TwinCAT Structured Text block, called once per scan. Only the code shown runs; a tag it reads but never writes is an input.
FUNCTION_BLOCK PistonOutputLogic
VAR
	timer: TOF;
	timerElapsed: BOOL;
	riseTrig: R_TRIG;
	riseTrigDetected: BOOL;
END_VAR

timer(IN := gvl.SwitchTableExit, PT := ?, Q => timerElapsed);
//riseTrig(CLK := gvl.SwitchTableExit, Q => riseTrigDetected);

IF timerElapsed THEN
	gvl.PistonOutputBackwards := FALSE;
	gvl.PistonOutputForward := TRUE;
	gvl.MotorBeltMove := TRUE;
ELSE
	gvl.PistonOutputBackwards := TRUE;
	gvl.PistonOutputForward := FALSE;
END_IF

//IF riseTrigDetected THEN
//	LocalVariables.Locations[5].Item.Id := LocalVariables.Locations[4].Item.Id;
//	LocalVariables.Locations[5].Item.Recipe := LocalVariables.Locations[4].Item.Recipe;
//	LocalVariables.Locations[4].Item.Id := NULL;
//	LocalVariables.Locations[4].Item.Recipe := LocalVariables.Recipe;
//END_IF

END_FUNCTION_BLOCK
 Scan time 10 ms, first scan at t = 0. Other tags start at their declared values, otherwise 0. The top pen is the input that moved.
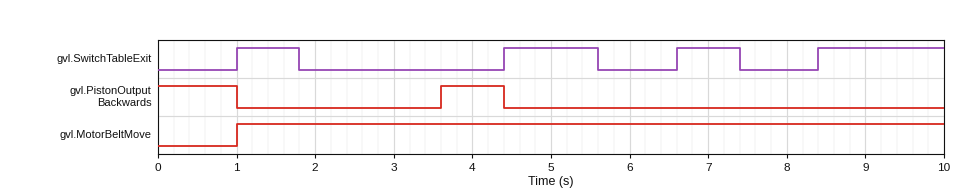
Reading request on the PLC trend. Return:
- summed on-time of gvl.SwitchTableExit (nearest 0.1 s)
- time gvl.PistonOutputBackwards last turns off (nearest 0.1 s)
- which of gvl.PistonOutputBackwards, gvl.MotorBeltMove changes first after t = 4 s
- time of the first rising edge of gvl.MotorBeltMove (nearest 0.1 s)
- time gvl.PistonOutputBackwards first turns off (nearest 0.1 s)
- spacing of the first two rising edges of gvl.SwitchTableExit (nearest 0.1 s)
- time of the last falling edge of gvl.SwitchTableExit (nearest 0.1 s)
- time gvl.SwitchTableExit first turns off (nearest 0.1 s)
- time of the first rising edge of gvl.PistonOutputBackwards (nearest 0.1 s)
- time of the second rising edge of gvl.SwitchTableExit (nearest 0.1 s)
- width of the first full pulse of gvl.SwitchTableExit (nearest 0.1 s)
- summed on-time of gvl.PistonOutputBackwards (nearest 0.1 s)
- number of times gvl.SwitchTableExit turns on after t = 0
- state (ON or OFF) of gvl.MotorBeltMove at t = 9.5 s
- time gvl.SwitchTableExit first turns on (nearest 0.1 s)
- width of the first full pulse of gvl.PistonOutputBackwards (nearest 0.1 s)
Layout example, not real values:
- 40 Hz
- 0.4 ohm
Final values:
- 4.4 s
- 4.4 s
- gvl.PistonOutputBackwards
- 1.0 s
- 1.0 s
- 3.4 s
- 7.4 s
- 1.8 s
- 3.6 s
- 4.4 s
- 0.8 s
- 1.8 s
- 4
- ON
- 1.0 s
- 0.8 s
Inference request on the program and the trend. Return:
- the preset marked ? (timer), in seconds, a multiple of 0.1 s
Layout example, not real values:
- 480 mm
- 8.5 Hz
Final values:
- 1.8 s
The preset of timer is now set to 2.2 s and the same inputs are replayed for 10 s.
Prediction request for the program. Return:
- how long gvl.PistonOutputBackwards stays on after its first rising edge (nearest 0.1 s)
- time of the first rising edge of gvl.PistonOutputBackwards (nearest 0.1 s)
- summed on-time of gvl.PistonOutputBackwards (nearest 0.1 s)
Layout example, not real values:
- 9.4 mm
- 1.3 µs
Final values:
- 0.4 s
- 4.0 s
- 1.4 s
